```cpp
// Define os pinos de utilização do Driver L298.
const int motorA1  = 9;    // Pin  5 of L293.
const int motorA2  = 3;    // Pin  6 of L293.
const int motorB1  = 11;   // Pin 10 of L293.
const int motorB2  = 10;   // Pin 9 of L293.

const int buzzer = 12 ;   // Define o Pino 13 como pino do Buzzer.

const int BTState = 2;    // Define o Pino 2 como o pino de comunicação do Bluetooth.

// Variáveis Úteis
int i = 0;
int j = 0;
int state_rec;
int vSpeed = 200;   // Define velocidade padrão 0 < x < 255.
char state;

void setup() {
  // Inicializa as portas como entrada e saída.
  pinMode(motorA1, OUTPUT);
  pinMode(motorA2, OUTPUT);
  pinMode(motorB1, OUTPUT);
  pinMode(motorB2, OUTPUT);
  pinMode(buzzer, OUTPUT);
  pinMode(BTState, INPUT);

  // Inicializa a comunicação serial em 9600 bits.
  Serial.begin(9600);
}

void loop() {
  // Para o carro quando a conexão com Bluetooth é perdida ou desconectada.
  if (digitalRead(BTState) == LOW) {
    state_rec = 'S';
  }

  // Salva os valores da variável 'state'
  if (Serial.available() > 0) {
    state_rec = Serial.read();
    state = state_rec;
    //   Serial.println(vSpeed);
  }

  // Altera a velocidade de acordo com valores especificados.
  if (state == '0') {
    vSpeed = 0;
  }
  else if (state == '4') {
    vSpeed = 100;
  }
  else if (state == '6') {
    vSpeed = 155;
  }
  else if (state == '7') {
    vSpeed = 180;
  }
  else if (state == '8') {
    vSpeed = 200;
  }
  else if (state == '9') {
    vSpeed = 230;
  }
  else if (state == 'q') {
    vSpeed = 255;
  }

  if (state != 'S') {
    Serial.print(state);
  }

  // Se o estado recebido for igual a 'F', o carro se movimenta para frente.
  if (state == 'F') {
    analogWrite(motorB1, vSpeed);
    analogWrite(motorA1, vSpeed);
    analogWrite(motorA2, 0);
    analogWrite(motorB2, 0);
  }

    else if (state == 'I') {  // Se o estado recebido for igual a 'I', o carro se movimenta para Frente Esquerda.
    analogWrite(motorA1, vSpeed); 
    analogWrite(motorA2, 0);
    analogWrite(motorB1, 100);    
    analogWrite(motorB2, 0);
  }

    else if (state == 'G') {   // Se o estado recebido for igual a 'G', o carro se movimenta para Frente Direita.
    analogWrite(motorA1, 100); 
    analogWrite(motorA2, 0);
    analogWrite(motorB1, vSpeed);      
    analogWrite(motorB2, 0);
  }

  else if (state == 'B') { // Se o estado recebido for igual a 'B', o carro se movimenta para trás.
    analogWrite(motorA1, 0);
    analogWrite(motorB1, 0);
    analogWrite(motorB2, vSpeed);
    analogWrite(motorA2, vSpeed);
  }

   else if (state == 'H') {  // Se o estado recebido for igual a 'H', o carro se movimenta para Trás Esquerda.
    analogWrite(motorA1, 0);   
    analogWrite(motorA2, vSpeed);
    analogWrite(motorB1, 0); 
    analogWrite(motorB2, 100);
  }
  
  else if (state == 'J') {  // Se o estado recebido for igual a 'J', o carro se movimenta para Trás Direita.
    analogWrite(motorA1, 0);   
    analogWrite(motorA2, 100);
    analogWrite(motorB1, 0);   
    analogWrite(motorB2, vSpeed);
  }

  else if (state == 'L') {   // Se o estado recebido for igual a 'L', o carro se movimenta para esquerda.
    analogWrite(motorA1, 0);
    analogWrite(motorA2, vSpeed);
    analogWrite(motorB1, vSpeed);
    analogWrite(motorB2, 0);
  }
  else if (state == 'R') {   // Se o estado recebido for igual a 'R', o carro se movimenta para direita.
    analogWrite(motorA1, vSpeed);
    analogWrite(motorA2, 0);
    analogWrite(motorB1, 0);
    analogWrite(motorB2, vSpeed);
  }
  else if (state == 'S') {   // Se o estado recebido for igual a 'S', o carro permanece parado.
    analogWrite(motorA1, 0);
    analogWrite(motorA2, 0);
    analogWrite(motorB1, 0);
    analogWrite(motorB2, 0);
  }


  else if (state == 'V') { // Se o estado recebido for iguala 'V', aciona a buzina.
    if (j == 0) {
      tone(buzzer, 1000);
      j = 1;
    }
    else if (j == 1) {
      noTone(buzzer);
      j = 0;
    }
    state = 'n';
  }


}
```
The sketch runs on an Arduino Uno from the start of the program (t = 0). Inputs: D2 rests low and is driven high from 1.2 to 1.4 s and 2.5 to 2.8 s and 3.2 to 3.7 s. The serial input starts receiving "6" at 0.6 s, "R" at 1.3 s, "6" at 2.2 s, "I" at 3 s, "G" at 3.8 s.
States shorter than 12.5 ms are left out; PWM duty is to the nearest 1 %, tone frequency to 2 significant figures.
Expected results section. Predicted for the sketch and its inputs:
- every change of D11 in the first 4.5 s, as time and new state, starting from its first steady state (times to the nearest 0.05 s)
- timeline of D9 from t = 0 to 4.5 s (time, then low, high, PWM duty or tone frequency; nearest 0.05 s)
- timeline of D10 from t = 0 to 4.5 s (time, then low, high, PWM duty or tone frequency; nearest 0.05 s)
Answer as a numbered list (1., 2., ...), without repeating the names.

1. 0 s low; 3 s PWM 39 %; 3.8 s PWM 61 %
2. 0 s low; 1.3 s PWM 61 %; 3.8 s PWM 39 %
3. 0 s low; 1.3 s PWM 61 %; 3 s low
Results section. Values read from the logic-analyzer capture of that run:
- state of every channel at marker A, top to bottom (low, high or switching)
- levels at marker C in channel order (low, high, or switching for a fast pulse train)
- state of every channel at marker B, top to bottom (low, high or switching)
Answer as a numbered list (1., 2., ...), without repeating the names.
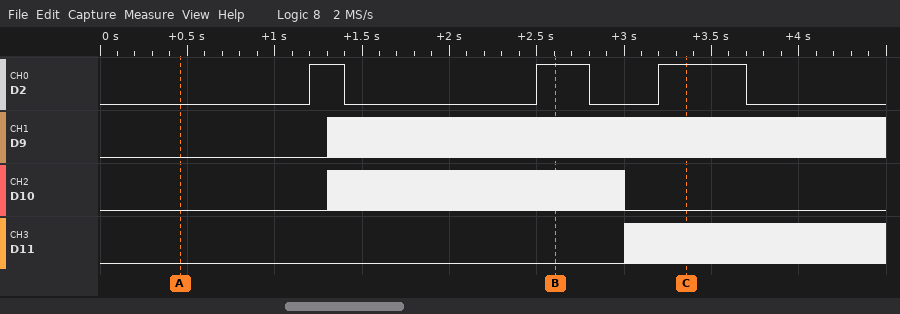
1. D2 low, D9 low, D10 low, D11 low
2. D2 high, D9 switching, D10 low, D11 switching
3. D2 high, D9 switching, D10 switching, D11 low
